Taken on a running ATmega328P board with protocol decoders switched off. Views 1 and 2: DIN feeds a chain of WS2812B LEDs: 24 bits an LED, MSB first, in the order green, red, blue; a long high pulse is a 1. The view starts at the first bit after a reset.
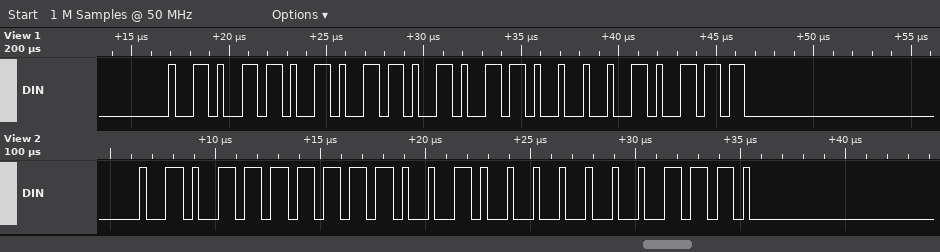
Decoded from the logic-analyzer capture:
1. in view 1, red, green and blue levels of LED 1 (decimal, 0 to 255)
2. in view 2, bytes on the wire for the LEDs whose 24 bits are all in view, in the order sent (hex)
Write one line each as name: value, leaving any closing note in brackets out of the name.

in view 1, red, green and blue levels of LED 1: 214, 90, 23
in view 2, bytes on the wire for the LEDs whose 24 bits are all in view, in the order sent: 5F C8 0E
